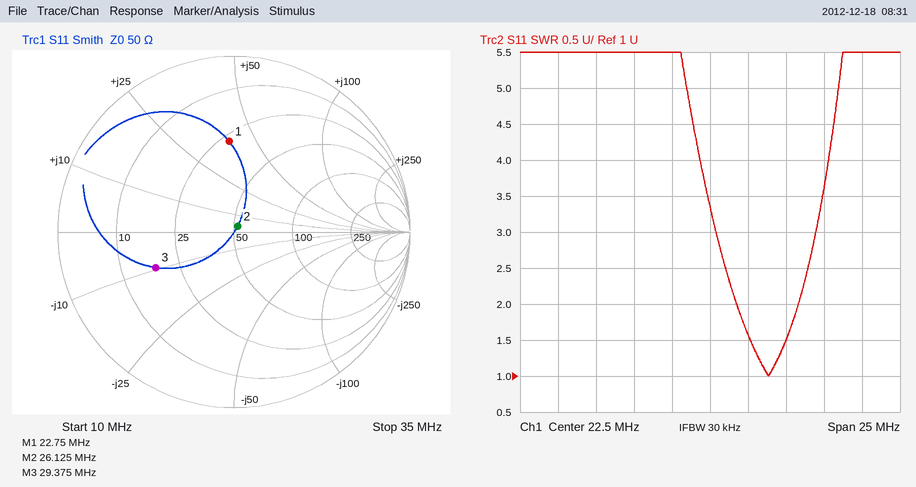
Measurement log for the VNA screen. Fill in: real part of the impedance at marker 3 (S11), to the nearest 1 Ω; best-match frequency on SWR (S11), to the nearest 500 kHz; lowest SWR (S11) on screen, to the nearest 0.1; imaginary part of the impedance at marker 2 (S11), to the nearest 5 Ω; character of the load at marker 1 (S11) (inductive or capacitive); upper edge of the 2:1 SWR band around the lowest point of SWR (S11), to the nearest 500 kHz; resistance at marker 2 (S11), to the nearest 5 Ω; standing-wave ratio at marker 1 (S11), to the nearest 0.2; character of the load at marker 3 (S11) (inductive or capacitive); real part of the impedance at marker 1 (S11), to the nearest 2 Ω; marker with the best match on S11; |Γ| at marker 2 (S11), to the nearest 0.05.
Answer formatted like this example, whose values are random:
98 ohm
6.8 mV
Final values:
18 Ω
26.5 MHz
1.0
+5 Ω
inductive
28.5 MHz
50 Ω
3.2
capacitive
28 Ω
marker 2
0.05
